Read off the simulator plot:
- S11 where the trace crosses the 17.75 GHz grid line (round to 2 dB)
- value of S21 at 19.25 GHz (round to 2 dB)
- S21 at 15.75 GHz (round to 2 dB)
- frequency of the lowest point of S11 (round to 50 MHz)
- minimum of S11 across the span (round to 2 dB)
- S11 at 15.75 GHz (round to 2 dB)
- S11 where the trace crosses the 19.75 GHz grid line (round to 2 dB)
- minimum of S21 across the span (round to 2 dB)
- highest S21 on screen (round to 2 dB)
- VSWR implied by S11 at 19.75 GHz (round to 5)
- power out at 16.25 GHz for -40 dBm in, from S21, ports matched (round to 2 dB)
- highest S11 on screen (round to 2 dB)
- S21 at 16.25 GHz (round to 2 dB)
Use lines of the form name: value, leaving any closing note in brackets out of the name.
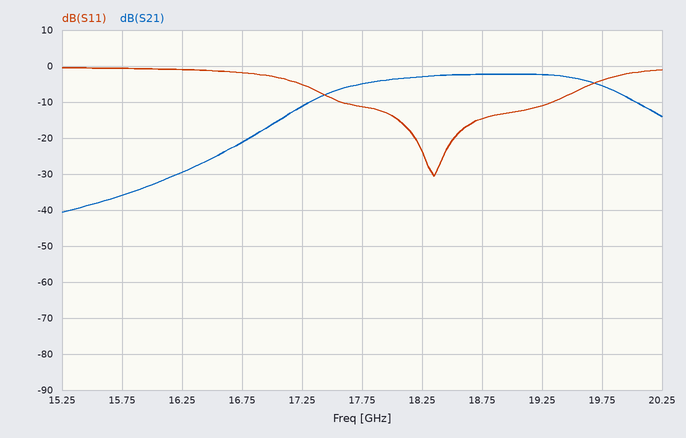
S11 where the trace crosses the 17.75 GHz grid line: -12 dB
value of S21 at 19.25 GHz: -2 dB
S21 at 15.75 GHz: -36 dB
frequency of the lowest point of S11: 18.35 GHz
minimum of S11 across the span: -30 dB
S11 at 15.75 GHz: 0 dB
S11 where the trace crosses the 19.75 GHz grid line: -4 dB
minimum of S21 across the span: -40 dB
highest S21 on screen: -2 dB
VSWR implied by S11 at 19.75 GHz: 5
power out at 16.25 GHz for -40 dBm in, from S21, ports matched: -70 dBm
highest S11 on screen: 0 dB
S21 at 16.25 GHz: -30 dB
